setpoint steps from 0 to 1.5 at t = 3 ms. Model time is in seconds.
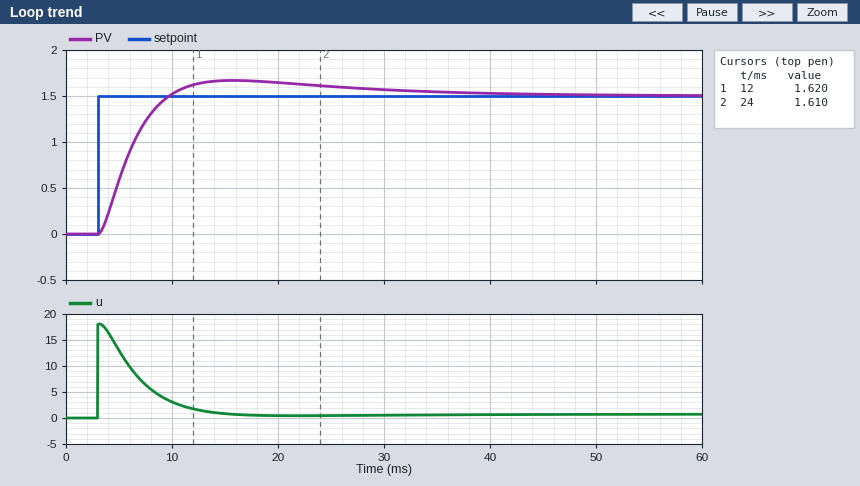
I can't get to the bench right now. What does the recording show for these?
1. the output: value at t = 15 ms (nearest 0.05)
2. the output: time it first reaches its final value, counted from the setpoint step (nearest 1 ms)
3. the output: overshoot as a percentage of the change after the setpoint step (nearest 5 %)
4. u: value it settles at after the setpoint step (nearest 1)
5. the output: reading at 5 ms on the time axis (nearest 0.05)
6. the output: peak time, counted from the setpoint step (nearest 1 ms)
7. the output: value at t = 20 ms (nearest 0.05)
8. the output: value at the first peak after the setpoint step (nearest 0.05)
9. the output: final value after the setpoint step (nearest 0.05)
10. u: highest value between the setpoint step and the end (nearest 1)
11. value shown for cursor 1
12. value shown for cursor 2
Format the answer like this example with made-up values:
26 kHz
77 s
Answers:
1.65
7 ms
10 %
1
0.60
13 ms
1.65
1.65
1.50
18
1.620
1.610
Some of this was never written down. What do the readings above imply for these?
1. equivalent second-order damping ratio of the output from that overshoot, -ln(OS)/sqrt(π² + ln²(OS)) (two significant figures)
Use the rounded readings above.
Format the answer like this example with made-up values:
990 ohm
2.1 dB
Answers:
0.59
